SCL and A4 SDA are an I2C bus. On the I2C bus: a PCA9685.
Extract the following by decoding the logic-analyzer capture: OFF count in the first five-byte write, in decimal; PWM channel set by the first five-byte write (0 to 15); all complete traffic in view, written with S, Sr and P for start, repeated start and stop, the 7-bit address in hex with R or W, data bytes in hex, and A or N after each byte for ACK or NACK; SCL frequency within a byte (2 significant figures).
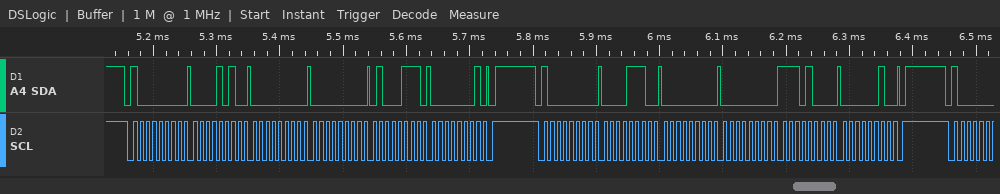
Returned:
327
1
S 40W A 0A A 00 A 00 A 47 A 01 A P S 40W A 0E A 00 A 00 A E8 A 02 A P
100 kHz
